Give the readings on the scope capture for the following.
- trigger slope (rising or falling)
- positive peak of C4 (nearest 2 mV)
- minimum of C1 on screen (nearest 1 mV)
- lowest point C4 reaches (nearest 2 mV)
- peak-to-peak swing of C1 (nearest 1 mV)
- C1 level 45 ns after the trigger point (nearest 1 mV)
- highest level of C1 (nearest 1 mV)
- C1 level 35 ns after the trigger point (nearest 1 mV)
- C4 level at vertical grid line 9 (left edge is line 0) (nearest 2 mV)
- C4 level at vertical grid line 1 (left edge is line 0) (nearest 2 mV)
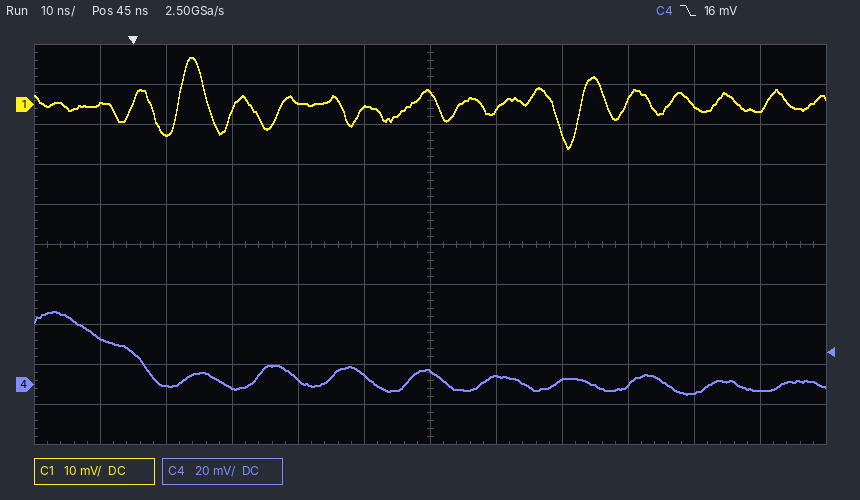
falling
36 mV
-11 mV
-4 mV
23 mV
3 mV
12 mV
-1 mV
0 mV
24 mV
